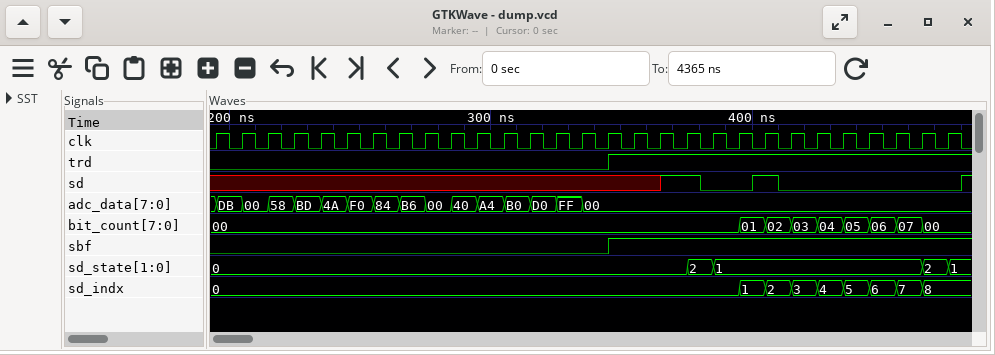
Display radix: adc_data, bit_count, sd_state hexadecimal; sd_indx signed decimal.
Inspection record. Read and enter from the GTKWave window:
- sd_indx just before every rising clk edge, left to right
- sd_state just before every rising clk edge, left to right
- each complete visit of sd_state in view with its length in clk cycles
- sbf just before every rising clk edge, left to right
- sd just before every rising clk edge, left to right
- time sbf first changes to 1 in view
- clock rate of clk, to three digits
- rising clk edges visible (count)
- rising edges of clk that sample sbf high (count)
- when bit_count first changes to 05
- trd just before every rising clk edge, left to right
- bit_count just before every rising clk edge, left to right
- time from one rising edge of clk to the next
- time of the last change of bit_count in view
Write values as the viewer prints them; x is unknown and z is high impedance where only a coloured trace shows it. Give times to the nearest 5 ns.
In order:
0, 0, 0, 0, 0, 0, 0, 0, 0, 0, 0, 0, 0, 0, 0, 0, 0, 0, 0, 0, 0, 1, 2, 3, 4, 5, 6, 7, 8
0, 0, 0, 0, 0, 0, 0, 0, 0, 0, 0, 0, 0, 0, 0, 0, 0, 0, 0, 2, 1, 1, 1, 1, 1, 1, 1, 1, 2
2: 1, 1: 8, 2: 1
0 0 0 0 0 0 0 0 0 0 0 0 0 0 0 0 1 1 1 1 1 1 1 1 1 1 1 1 1
x x x x x x x x x x x x x x x x x x 1 0 0 1 0 0 0 0 0 0 0
345 ns
100 MHz
29
13
435 ns
0 0 0 0 0 0 0 0 0 0 0 0 0 0 0 0 1 1 1 1 1 1 1 1 1 1 1 1 1
00, 00, 00, 00, 00, 00, 00, 00, 00, 00, 00, 00, 00, 00, 00, 00, 00, 00, 00, 00, 00, 01, 02, 03, 04, 05, 06, 07, 00
10 ns
465 ns
